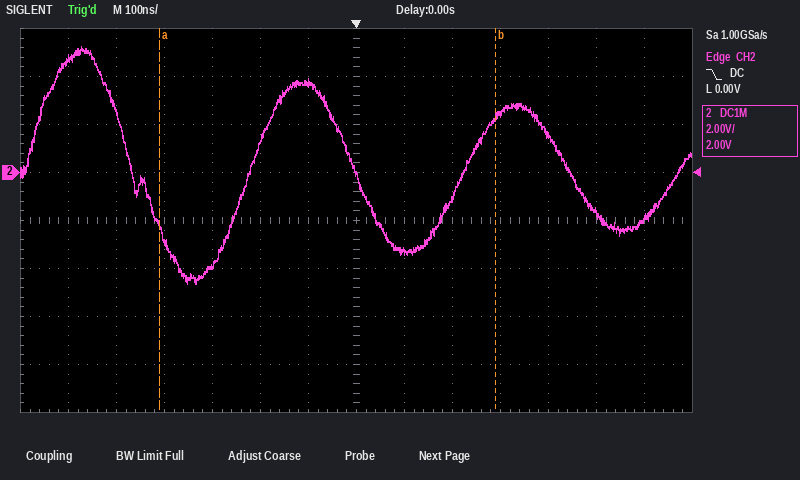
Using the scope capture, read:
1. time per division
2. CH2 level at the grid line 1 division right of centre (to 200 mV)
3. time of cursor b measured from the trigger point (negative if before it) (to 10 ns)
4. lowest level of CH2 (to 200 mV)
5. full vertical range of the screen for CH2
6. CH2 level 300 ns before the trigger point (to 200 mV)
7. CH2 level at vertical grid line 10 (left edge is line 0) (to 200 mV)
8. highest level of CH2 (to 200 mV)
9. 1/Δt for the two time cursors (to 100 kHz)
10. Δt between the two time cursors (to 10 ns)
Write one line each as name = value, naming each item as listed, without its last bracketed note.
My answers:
time per division = 100 ns
CH2 level at the grid line 1 division right of centre = -3.2 V
time of cursor b measured from the trigger point (negative if before it) = +290 ns
lowest level of CH2 = -4.6 V
full vertical range of the screen for CH2 = 16 V
CH2 level 300 ns before the trigger point = -3.8 V
CH2 level at vertical grid line 10 (left edge is line 0) = 2.4 V
highest level of CH2 = 5.2 V
1/Δt for the two time cursors = 1.4 MHz
Δt between the two time cursors = 700 ns
